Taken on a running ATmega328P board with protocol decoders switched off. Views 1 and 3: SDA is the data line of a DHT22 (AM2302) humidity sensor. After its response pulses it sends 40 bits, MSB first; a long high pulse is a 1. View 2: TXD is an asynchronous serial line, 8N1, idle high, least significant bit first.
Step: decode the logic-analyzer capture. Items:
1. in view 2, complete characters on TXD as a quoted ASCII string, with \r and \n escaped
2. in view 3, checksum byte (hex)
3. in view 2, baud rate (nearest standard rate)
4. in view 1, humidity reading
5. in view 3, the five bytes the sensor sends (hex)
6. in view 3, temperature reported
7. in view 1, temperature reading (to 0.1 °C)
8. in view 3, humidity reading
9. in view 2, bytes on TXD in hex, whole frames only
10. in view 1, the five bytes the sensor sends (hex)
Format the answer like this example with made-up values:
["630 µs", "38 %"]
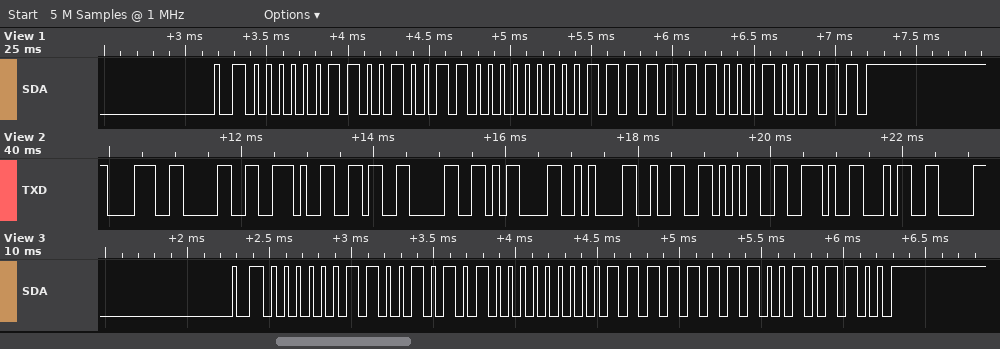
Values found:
["\"80.60\\r\\n25.4\"", "0x2C", "9600 baud", "80.6 %", "03 2A 00 FF 2C", "25.5 °C", "25.4 °C", "81.0 %", "38 30 2E 36 30 0D 0A 32 35 2E 34", "03 26 00 FE 27"]
